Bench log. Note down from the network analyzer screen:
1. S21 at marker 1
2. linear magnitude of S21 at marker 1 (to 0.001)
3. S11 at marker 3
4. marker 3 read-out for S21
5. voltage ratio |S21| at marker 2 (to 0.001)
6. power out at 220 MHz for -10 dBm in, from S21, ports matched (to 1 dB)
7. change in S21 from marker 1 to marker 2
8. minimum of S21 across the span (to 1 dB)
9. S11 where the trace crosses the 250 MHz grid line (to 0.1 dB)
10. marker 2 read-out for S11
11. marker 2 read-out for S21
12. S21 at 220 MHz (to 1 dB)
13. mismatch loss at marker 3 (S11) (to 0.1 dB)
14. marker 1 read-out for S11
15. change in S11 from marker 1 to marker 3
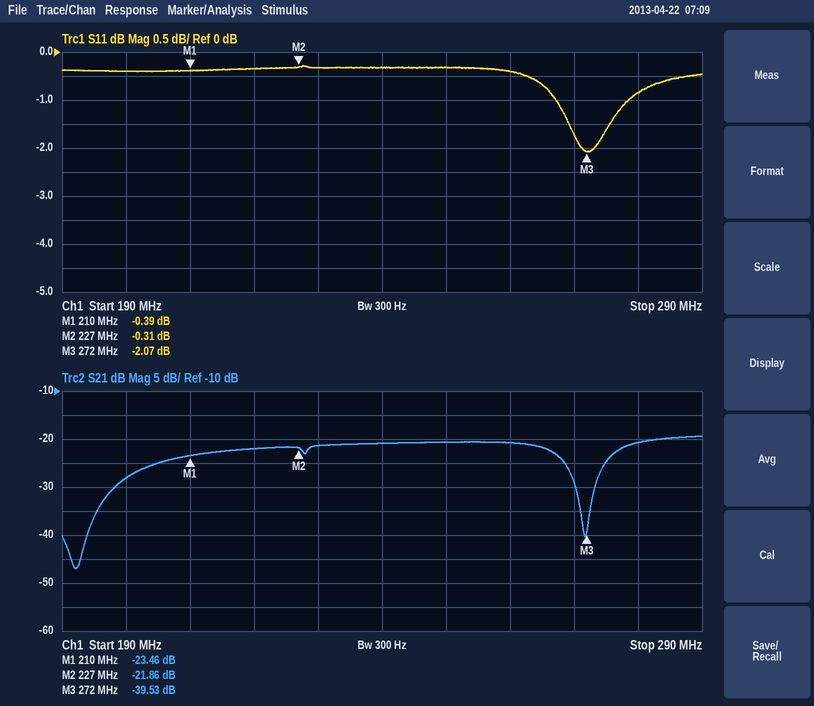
-23.46 dB
0.067
-2.07 dB
-39.53 dB
0.081
-32 dBm
1.60 dB
-47 dB
-0.3 dB
-0.31 dB
-21.86 dB
-22 dB
4.2 dB
-0.39 dB
-1.68 dB
